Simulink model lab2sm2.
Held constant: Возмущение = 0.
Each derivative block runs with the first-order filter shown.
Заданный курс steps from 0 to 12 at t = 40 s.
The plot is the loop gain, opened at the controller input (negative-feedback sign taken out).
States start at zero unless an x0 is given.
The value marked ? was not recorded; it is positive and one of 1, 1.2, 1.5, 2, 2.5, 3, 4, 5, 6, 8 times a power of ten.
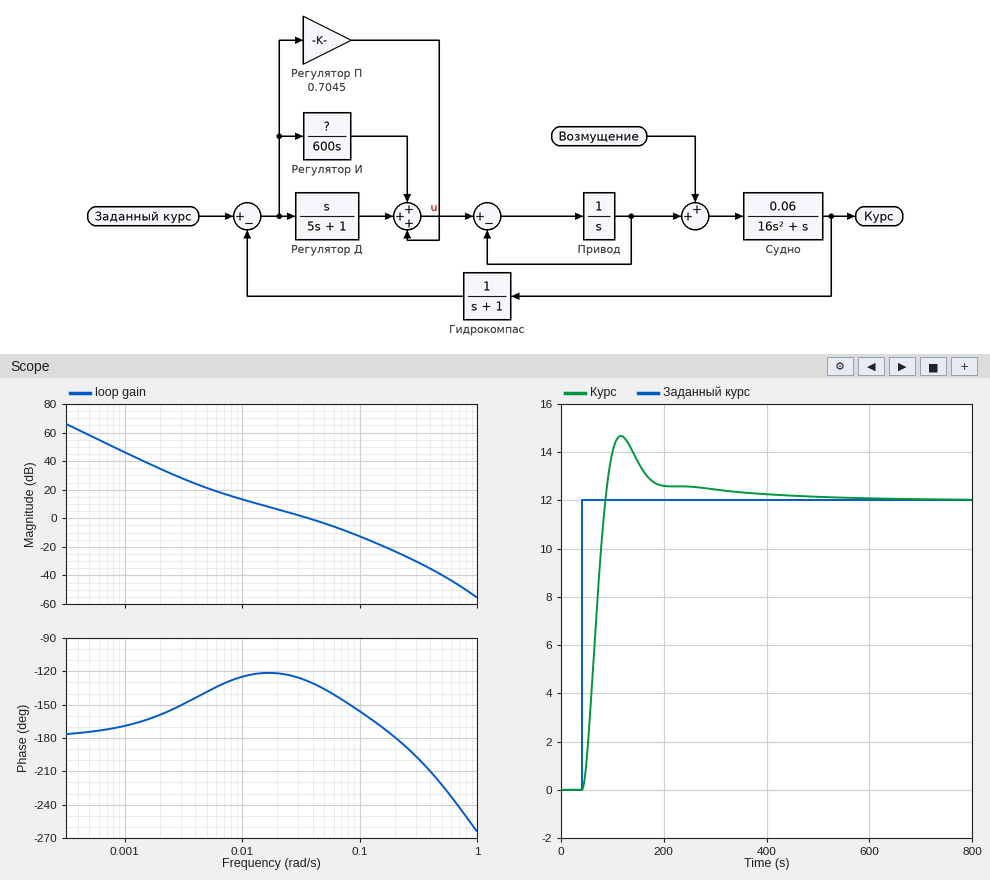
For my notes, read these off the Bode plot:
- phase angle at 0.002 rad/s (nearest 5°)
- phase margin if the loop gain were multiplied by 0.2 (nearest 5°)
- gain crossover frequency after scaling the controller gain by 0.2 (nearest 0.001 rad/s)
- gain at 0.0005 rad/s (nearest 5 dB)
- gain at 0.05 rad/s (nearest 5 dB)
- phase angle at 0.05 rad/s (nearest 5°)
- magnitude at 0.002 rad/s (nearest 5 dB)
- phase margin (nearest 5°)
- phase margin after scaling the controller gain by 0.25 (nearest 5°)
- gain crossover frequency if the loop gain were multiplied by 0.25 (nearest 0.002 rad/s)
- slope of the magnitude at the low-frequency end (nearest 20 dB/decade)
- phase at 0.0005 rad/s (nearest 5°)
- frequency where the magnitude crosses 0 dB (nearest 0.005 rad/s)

-160°
55°
0.009 rad/s
60 dB
-5 dB
-135°
35 dB
50°
55°
0.012 rad/s
-40 dB/decade
-175°
0.035 rad/s
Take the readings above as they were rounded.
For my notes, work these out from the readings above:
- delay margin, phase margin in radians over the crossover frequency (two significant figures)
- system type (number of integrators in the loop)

25 s
2
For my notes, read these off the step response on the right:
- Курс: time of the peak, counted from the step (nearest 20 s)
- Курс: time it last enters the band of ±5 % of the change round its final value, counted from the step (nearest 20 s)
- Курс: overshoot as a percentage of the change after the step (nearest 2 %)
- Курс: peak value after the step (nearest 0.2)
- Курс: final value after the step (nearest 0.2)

80 s
160 s
22 %
14.6
12.0
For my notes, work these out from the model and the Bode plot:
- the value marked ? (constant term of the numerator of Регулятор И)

2
